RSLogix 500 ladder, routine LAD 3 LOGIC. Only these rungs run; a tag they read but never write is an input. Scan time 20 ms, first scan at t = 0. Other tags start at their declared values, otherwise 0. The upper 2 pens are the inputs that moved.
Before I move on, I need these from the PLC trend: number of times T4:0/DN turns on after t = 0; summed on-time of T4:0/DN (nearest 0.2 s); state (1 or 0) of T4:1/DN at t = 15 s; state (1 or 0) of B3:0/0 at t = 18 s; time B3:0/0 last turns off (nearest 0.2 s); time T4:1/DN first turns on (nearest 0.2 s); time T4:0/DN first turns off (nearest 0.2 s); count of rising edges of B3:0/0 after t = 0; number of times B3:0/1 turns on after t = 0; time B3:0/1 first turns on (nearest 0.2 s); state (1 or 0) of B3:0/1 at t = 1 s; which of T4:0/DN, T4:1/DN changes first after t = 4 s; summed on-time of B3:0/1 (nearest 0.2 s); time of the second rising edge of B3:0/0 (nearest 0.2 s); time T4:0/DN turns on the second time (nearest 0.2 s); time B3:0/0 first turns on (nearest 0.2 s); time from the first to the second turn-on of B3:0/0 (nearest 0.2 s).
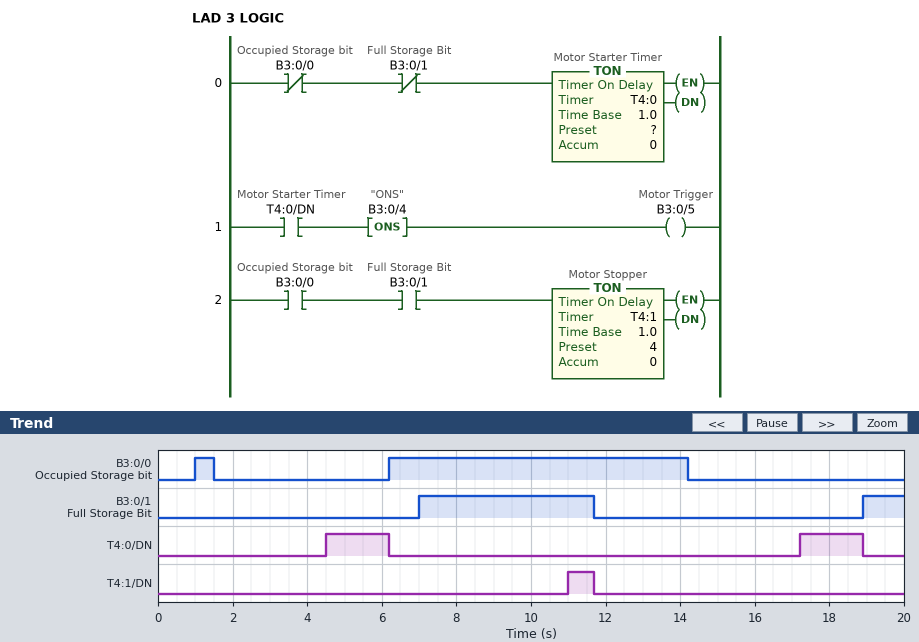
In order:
2
3.4 s
0
0
14.2 s
11.0 s
6.2 s
2
2
7.0 s
0
T4:0/DN
5.8 s
6.2 s
17.2 s
1.0 s
5.2 s
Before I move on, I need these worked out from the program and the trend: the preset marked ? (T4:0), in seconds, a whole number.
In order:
3 s
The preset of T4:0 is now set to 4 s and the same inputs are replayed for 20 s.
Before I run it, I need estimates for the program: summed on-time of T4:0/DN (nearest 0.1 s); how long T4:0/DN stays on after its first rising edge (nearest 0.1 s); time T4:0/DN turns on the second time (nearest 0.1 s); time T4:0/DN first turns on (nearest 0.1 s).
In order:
1.4 s
0.7 s
18.2 s
5.5 s
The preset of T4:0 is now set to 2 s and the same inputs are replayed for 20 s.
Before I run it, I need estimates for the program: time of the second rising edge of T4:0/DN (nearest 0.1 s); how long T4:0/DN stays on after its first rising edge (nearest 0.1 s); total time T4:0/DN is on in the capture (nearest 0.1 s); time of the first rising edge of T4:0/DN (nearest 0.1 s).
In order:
16.2 s
2.7 s
5.4 s
3.5 s
